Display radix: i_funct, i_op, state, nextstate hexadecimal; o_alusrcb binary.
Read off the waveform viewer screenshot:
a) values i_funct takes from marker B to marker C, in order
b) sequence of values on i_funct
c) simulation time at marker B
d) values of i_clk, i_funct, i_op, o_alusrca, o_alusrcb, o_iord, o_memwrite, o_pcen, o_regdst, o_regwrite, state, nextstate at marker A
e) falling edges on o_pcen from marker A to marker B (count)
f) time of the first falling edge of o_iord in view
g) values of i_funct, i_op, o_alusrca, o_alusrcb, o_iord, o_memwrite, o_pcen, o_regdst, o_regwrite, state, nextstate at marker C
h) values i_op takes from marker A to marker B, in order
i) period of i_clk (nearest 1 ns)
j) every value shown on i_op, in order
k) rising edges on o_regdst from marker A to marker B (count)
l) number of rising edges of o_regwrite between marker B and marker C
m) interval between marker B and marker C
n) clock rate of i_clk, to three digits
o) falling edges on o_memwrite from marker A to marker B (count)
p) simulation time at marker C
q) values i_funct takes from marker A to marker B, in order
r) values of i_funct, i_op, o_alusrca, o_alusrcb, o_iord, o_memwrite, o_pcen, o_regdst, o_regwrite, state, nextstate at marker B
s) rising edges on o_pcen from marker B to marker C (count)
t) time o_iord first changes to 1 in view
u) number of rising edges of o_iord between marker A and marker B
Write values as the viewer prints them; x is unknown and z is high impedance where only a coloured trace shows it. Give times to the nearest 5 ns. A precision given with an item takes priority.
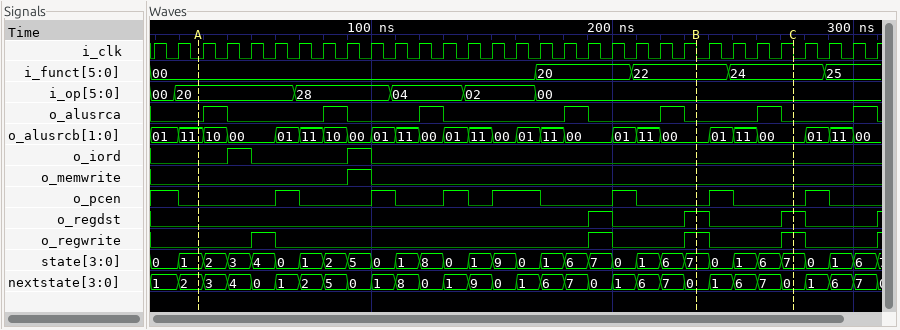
22, 24
00, 20, 22, 24, 25
235 ns
i_clk=0, i_funct=00, i_op=20, o_alusrca=0, o_alusrcb=11, o_iord=0, o_memwrite=0, o_pcen=0, o_regdst=0, o_regwrite=0, state=1, nextstate=2
5
50 ns
i_funct=24, i_op=00, o_alusrca=0, o_alusrcb=00, o_iord=0, o_memwrite=0, o_pcen=0, o_regdst=1, o_regwrite=1, state=7, nextstate=0
20, 28, 04, 02, 00
10 ns
00, 20, 28, 04, 02, 00
2
1
40 ns
100 MHz
1
275 ns
00, 20, 22
i_funct=22, i_op=00, o_alusrca=0, o_alusrcb=00, o_iord=0, o_memwrite=0, o_pcen=0, o_regdst=1, o_regwrite=1, state=7, nextstate=0
1
40 ns
2
